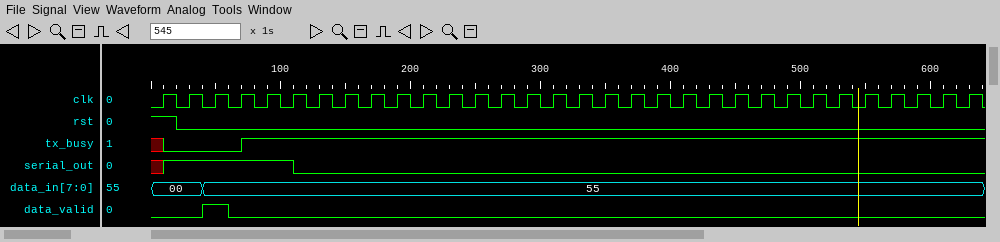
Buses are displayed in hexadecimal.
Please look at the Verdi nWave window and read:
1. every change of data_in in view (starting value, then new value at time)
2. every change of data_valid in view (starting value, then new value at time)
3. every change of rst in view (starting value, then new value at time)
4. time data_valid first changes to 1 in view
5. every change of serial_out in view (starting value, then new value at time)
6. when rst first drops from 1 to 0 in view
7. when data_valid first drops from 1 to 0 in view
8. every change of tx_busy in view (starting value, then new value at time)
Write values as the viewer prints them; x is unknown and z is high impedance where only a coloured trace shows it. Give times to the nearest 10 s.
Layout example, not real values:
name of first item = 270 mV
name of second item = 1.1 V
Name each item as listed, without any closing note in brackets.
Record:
every change of data_in in view = 00, 55 at 40 s
every change of data_valid in view = 0, 1 at 40 s, 0 at 60 s
every change of rst in view = 1, 0 at 20 s
time data_valid first changes to 1 in view = 40 s
every change of serial_out in view = x, 1 at 10 s, 0 at 110 s
when rst first drops from 1 to 0 in view = 20 s
when data_valid first drops from 1 to 0 in view = 60 s
every change of tx_busy in view = x, 0 at 10 s, 1 at 70 s
